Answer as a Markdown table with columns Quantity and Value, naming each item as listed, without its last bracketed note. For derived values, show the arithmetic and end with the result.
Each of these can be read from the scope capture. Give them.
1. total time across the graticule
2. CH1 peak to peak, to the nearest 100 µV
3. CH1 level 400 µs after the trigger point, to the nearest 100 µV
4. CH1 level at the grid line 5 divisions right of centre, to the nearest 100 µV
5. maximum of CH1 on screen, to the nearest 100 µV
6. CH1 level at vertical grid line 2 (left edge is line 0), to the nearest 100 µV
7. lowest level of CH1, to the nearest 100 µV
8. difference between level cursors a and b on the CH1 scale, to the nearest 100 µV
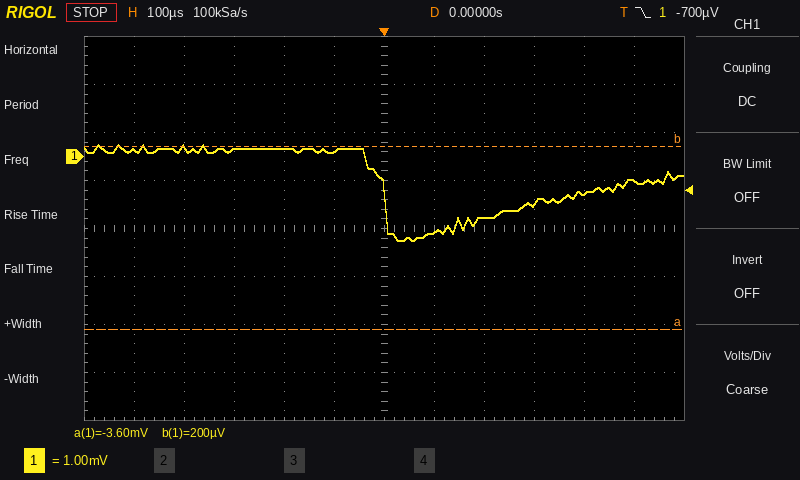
| Quantity | Value |
|---|---|
| total time across the graticule | 1.2 ms |
| CH1 peak to peak, to the nearest 100 µV | 200 µV − (-1.8 mV) = 2.0 mV |
| CH1 level 400 µs after the trigger point, to the nearest 100 µV | -800 µV |
| CH1 level at the grid line 5 divisions right of centre, to the nearest 100 µV | -500 µV |
| maximum of CH1 on screen, to the nearest 100 µV | 200 µV |
| CH1 level at vertical grid line 2 (left edge is line 0), to the nearest 100 µV | 200 µV |
| lowest level of CH1, to the nearest 100 µV | -1.8 mV |
| difference between level cursors a and b on the CH1 scale, to the nearest 100 µV | 3.8 mV |
